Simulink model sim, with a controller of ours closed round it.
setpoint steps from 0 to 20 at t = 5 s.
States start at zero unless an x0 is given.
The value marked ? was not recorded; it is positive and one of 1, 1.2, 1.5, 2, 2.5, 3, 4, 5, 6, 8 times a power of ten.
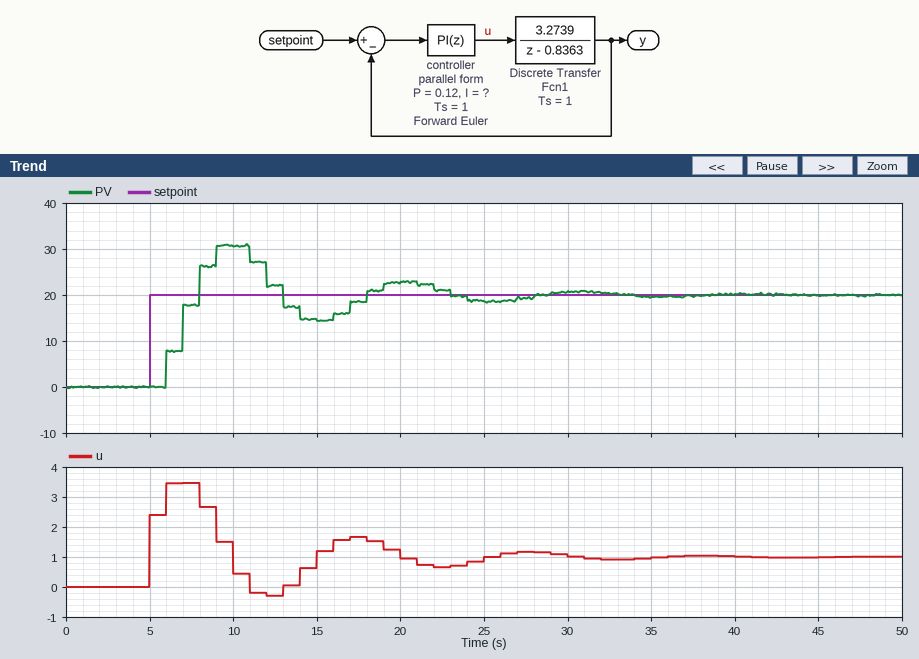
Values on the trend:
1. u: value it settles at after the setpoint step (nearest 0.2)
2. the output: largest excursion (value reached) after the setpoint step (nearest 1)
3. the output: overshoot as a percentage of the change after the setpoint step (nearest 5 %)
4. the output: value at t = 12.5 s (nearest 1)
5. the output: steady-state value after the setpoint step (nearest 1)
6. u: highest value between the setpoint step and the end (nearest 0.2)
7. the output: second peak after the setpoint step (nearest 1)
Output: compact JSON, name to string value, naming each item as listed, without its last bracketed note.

{"u: value it settles at after the setpoint step": "1.0", "the output: largest excursion (value reached) after the setpoint step": "31", "the output: overshoot as a percentage of the change after the setpoint step": "55 %", "the output: value at t = 12.5 s": "22", "the output: steady-state value after the setpoint step": "20", "u: highest value between the setpoint step and the end": "3.4", "the output: second peak after the setpoint step": "23"}
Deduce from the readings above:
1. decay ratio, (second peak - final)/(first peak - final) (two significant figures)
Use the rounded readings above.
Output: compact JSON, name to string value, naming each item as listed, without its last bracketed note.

{"decay ratio, (second peak - final)/(first peak - final)": "0.27"}
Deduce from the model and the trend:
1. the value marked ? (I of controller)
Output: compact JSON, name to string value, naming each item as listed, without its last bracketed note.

{"the value marked ?": "0.1"}
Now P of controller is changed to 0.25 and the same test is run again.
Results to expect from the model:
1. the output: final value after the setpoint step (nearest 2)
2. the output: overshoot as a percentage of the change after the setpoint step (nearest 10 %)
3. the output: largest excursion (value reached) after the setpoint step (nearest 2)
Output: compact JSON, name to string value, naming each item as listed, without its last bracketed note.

{"the output: final value after the setpoint step": "20", "the output: overshoot as a percentage of the change after the setpoint step": "20 %", "the output: largest excursion (value reached) after the setpoint step": "24"}
